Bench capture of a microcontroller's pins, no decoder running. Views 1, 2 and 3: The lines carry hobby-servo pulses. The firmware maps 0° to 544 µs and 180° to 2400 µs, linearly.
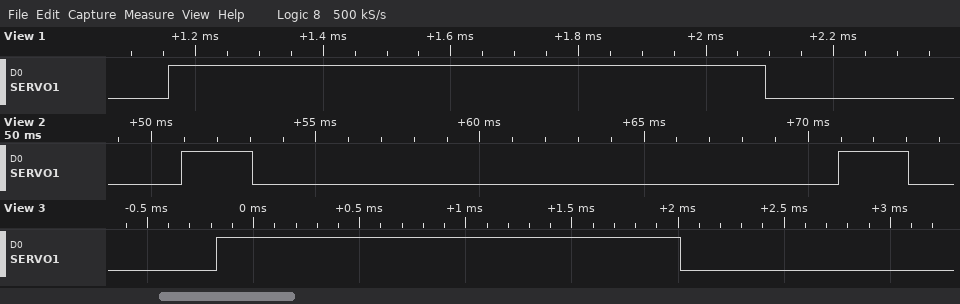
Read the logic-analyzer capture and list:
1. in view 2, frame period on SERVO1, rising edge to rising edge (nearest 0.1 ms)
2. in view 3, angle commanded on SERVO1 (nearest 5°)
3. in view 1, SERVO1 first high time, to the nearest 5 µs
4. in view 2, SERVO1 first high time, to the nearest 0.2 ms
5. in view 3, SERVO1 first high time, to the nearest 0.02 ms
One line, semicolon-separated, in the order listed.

20.0 ms; 160°; 935 µs; 2.2 ms; 2.18 ms
